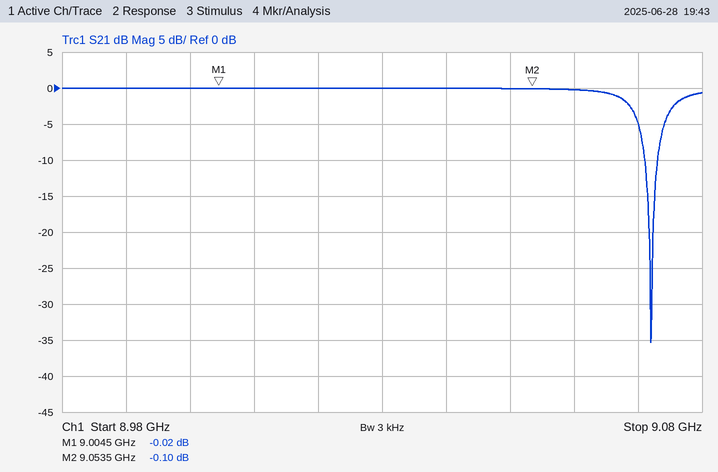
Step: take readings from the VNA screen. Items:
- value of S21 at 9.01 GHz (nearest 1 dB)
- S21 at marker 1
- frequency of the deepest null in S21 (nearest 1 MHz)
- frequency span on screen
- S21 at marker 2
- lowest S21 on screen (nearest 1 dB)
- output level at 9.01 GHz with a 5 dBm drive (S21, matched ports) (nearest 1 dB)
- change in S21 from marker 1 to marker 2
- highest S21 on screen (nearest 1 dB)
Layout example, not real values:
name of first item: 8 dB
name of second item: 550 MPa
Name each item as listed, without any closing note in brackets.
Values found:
value of S21 at 9.01 GHz: 0 dB
S21 at marker 1: -0.02 dB
frequency of the deepest null in S21: 9.072 GHz
frequency span on screen: 100 MHz
S21 at marker 2: -0.10 dB
lowest S21 on screen: -35 dB
output level at 9.01 GHz with a 5 dBm drive (S21, matched ports): 5 dBm
change in S21 from marker 1 to marker 2: -0.08 dB
highest S21 on screen: 0 dB
